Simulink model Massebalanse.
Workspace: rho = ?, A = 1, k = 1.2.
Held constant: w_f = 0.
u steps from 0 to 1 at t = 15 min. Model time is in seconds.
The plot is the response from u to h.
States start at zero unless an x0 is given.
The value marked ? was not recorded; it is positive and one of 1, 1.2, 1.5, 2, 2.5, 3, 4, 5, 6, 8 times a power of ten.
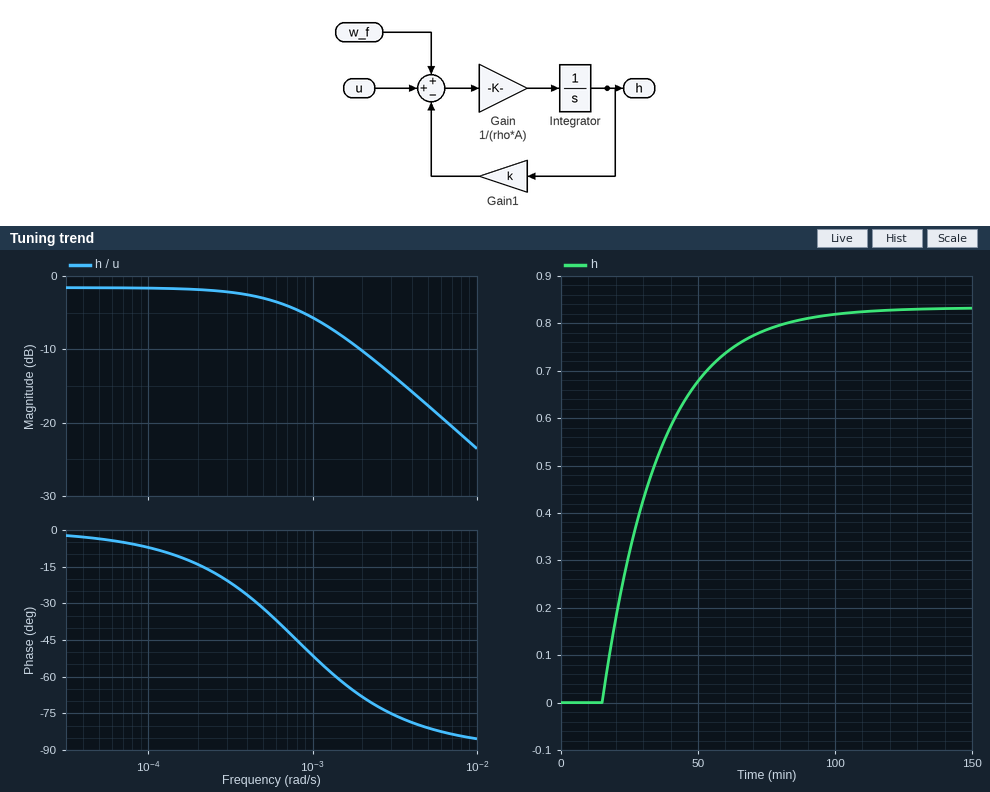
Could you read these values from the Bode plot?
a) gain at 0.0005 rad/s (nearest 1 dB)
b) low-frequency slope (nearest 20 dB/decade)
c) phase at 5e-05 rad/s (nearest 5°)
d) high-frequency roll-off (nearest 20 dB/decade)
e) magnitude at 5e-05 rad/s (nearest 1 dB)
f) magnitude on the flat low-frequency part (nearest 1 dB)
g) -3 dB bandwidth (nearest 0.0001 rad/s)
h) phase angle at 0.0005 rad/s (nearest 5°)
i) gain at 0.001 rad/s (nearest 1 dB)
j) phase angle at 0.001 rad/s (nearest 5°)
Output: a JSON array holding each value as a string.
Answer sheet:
["-3 dB", "0 dB/decade", "-5°", "-20 dB/decade", "-2 dB", "-2 dB", "0.0008 rad/s", "-30°", "-6 dB", "-50°"]
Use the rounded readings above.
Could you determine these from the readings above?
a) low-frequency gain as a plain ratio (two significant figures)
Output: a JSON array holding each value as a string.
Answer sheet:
["0.79"]
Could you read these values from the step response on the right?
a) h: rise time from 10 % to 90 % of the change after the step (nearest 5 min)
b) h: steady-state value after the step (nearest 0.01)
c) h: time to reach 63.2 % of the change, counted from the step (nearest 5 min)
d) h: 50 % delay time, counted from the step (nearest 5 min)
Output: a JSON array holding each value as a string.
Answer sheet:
["45 min", "0.83", "20 min", "15 min"]
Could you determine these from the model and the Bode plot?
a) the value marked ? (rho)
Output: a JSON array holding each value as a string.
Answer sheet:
["1500"]
